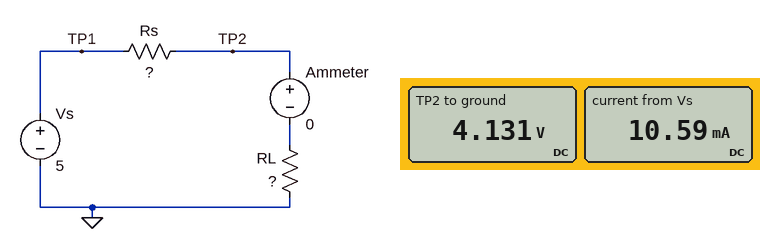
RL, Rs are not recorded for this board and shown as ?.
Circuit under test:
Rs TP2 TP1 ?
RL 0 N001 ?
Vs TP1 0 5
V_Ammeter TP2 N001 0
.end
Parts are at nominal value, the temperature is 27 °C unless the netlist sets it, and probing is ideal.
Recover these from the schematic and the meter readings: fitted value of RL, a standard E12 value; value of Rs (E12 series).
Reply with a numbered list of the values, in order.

1. 390 Ω
2. 82 Ω
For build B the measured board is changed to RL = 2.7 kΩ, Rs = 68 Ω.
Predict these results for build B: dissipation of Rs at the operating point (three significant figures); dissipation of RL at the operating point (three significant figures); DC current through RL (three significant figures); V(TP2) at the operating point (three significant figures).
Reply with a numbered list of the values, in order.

1. 222 µW
2. 8.81 mW
3. 1.81 mA
4. 4.88 V
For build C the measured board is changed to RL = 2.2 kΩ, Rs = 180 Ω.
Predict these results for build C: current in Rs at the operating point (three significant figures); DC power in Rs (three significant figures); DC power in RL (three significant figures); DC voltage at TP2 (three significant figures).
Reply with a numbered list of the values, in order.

1. 2.10 mA
2. 794 µW
3. 9.71 mW
4. 4.62 V
